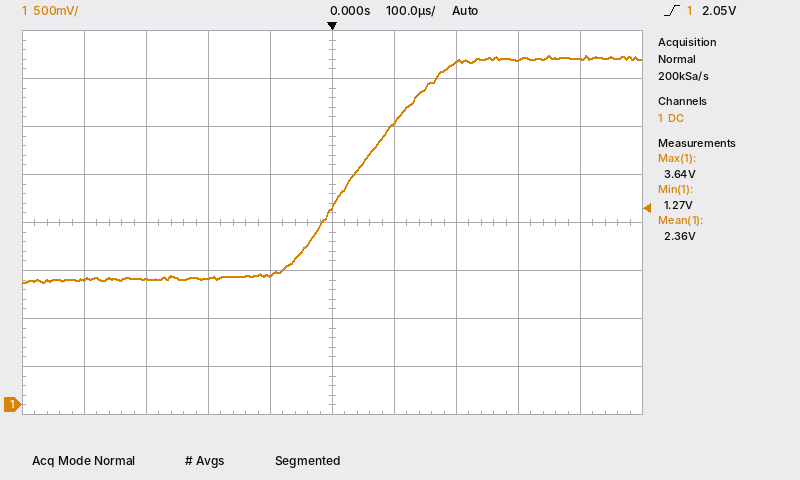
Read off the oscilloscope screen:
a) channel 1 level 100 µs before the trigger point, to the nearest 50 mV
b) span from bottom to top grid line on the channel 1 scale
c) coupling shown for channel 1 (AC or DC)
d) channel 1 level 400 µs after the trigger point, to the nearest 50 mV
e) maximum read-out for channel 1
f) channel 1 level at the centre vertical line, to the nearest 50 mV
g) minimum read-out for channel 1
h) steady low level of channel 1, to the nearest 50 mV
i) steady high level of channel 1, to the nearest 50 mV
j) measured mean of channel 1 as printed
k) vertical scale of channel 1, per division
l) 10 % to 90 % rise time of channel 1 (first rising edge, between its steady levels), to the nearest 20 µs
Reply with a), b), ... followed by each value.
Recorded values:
a) 1.35 V
b) 4 V
c) DC
d) 3.60 V
e) 3.64 V
f) 2.05 V
g) 1.27 V
h) 1.30 V
i) 3.60 V
j) 2.36 V
k) 500 mV
l) 220 µs
